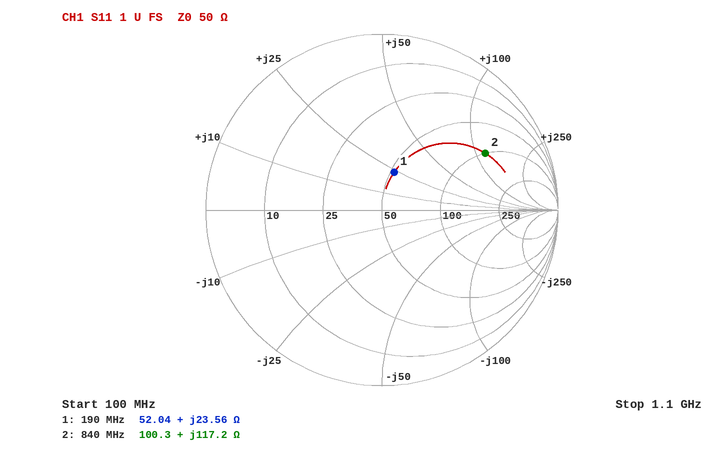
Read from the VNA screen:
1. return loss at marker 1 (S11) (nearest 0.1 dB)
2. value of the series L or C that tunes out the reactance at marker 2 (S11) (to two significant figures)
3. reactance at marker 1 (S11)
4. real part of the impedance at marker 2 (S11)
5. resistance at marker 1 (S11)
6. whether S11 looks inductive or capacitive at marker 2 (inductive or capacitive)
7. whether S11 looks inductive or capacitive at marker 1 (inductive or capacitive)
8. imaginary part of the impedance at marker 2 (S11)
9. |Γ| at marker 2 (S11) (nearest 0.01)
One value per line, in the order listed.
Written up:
12.9 dB
1.6 pF
+23.56 Ω
100.3 Ω
52.04 Ω
inductive
inductive
+117.2 Ω
0.67
